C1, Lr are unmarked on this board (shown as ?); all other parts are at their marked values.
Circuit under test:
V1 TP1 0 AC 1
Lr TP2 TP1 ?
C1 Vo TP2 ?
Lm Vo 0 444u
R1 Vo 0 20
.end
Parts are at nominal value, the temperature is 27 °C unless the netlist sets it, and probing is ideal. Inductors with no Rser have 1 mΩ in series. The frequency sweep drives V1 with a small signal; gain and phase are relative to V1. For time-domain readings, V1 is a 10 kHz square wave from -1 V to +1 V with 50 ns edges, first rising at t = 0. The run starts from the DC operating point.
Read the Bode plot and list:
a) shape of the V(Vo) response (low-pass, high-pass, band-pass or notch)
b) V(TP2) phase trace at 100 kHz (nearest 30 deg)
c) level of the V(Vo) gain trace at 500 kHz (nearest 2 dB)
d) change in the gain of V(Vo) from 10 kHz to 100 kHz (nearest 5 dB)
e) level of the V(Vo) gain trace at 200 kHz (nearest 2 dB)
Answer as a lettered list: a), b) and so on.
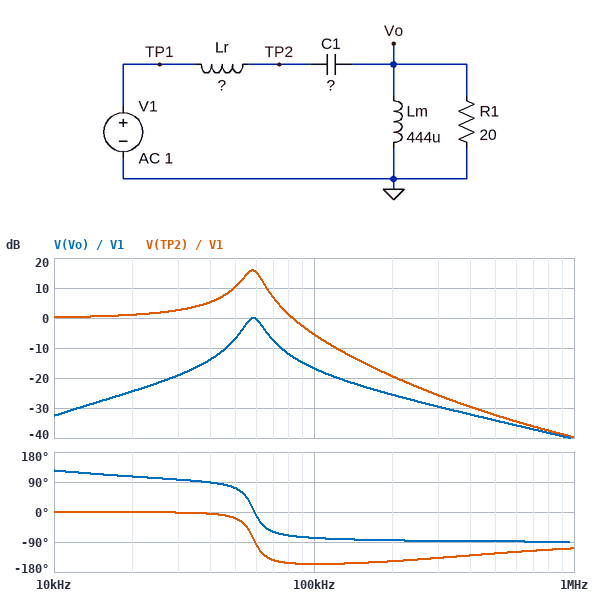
a) band-pass
b) -150 deg
c) -34 dB
d) 15 dB
e) -26 dB
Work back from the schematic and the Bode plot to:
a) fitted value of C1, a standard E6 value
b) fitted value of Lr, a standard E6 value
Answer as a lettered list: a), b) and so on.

a) 22 nF
b) 330 µH
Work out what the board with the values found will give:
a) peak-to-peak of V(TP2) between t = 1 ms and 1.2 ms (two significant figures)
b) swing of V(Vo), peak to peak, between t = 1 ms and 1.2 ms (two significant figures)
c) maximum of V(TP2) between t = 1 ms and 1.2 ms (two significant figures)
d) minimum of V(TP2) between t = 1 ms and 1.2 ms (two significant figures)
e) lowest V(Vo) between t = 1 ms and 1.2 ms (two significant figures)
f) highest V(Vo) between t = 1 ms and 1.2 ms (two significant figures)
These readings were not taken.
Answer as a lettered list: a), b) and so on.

a) 4.6 V
b) 430 mV
c) 2.3 V
d) -2.3 V
e) -220 mV
f) 220 mV
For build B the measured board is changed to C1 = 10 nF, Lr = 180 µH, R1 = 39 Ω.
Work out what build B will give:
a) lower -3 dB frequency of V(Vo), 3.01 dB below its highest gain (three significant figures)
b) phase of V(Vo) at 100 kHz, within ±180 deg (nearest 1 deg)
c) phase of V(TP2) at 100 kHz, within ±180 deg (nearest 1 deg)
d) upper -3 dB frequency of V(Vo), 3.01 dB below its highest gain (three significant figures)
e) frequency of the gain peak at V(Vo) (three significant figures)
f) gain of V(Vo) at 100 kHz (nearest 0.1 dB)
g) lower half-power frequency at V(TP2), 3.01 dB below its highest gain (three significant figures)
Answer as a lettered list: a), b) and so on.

a) 101 kHz
b) 55 deg
c) -29 deg
d) 135 kHz
e) 117 kHz
f) -3.2 dB
g) 95.8 kHz
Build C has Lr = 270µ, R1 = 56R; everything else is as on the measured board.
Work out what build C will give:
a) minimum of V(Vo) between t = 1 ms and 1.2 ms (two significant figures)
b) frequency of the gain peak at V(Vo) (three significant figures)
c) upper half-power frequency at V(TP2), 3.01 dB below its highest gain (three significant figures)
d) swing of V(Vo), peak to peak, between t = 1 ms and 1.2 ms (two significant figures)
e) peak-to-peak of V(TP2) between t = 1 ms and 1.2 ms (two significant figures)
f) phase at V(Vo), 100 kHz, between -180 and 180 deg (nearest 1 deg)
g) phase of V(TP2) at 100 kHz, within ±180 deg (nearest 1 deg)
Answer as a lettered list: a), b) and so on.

a) -580 mV
b) 60.2 kHz
c) 70.9 kHz
d) 1.2 V
e) 4.0 V
f) -52 deg
g) -112 deg
